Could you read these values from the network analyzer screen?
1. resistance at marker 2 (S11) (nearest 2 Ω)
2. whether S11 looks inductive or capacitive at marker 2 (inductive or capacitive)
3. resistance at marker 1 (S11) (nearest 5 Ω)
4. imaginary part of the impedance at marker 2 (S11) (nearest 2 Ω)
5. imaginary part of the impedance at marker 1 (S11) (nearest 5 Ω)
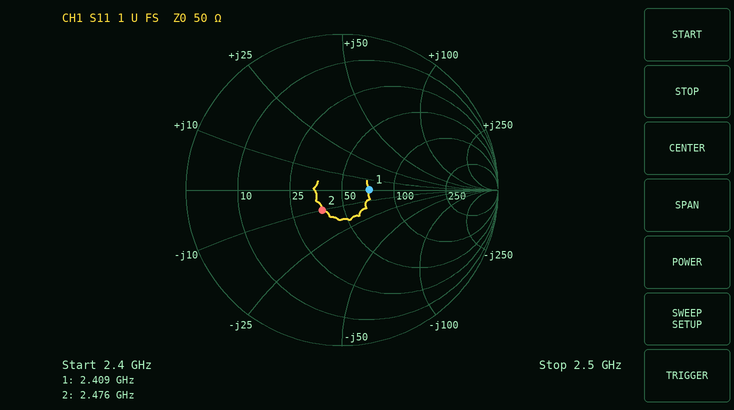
38 Ω
capacitive
70 Ω
-10 Ω
0 Ω
